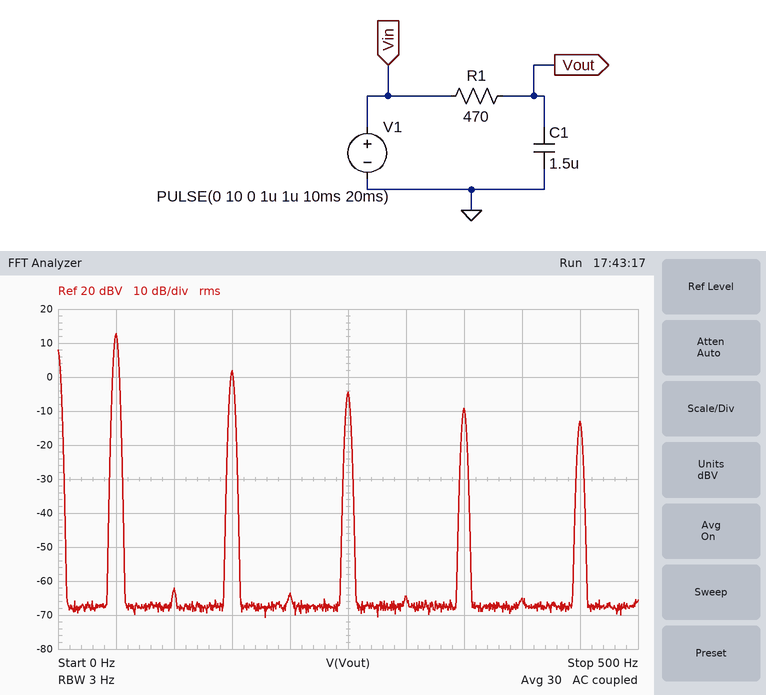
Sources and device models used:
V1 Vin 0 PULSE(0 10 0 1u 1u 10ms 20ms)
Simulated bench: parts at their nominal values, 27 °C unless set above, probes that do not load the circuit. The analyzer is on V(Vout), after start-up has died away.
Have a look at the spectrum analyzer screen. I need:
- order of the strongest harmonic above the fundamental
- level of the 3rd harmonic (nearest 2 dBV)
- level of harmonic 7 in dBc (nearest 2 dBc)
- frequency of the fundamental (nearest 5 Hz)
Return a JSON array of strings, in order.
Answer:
["3", "2 dBV", "-22 dBc", "50 Hz"]
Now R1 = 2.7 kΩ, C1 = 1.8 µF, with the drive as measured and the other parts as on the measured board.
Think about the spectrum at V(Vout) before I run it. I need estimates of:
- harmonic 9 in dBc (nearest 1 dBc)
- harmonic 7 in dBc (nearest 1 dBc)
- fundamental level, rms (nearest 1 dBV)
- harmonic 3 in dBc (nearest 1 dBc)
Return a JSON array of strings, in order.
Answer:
["-37 dBc", "-32 dBc", "8 dBV", "-18 dBc"]
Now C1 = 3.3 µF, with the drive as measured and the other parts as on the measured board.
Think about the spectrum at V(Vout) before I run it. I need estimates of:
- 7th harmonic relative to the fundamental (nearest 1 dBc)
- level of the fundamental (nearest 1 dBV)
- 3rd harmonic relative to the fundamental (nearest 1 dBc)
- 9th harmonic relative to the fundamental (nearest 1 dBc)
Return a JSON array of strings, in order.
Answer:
["-27 dBc", "12 dBV", "-14 dBc", "-31 dBc"]
